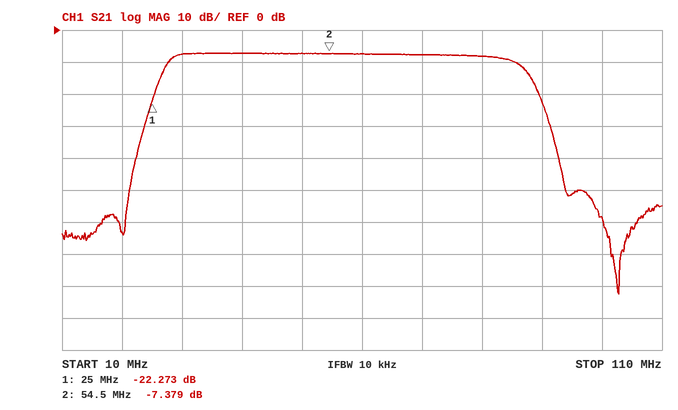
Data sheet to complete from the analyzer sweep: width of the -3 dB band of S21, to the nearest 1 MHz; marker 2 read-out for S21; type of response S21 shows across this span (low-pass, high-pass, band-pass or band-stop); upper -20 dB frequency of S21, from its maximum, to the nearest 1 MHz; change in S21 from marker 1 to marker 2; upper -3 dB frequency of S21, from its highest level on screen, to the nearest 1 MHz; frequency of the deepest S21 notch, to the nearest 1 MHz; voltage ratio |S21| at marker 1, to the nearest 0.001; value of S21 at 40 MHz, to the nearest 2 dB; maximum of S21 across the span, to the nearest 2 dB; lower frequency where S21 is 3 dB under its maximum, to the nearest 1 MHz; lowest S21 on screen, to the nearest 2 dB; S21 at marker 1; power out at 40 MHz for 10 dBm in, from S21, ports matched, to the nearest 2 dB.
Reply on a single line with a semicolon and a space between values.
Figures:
58 MHz; -7.379 dB; band-pass; 91 MHz; 14.894 dB; 86 MHz; 103 MHz; 0.077; -8 dB; -8 dB; 28 MHz; -82 dB; -22.273 dB; 2 dBm
